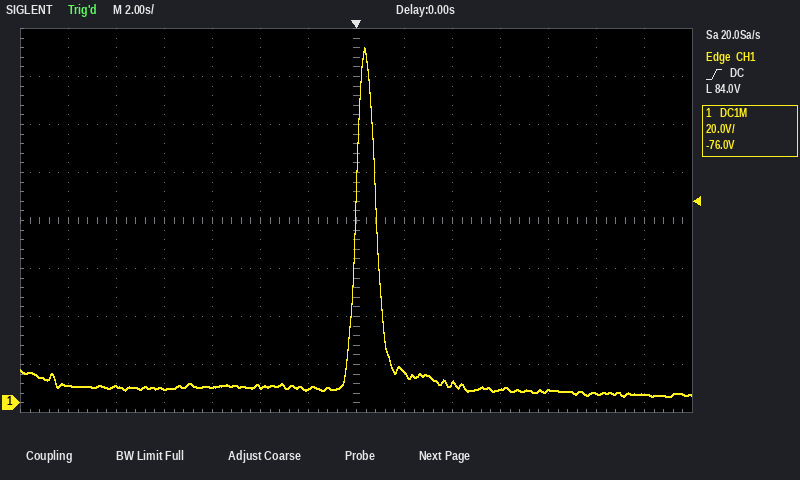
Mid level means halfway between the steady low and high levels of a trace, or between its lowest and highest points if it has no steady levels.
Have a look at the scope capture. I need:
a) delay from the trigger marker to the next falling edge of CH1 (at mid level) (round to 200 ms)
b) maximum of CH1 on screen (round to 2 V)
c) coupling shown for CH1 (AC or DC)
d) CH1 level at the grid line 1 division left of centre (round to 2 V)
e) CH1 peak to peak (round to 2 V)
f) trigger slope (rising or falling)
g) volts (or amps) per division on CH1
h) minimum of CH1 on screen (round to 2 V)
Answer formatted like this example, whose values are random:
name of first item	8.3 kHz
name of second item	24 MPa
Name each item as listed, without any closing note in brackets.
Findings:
delay from the trigger marker to the next falling edge of CH1 (at mid level)	800 ms
maximum of CH1 on screen	148 V
coupling shown for CH1	DC
CH1 level at the grid line 1 division left of centre	6 V
CH1 peak to peak	146 V
trigger slope	rising
volts (or amps) per division on CH1	20 V
minimum of CH1 on screen	2 V
